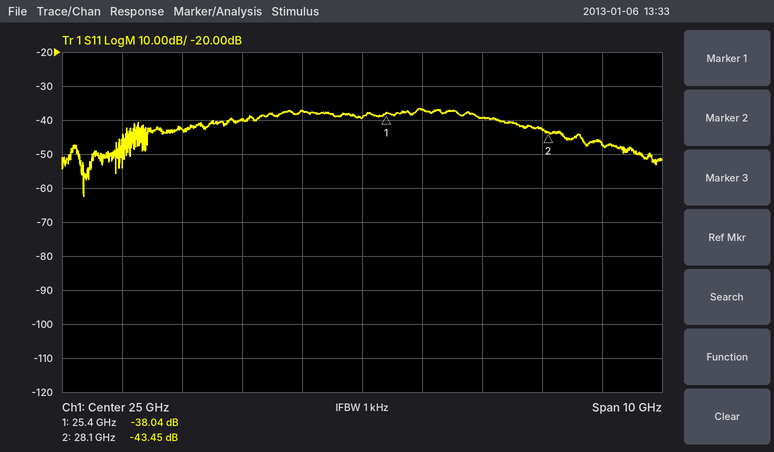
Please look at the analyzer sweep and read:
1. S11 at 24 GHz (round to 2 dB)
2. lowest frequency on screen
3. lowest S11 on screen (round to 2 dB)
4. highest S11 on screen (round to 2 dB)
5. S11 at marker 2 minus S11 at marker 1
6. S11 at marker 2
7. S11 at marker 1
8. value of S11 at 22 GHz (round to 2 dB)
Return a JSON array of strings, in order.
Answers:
["-38 dB", "20 GHz", "-62 dB", "-36 dB", "-5.41 dB", "-43.45 dB", "-38.04 dB", "-42 dB"]
